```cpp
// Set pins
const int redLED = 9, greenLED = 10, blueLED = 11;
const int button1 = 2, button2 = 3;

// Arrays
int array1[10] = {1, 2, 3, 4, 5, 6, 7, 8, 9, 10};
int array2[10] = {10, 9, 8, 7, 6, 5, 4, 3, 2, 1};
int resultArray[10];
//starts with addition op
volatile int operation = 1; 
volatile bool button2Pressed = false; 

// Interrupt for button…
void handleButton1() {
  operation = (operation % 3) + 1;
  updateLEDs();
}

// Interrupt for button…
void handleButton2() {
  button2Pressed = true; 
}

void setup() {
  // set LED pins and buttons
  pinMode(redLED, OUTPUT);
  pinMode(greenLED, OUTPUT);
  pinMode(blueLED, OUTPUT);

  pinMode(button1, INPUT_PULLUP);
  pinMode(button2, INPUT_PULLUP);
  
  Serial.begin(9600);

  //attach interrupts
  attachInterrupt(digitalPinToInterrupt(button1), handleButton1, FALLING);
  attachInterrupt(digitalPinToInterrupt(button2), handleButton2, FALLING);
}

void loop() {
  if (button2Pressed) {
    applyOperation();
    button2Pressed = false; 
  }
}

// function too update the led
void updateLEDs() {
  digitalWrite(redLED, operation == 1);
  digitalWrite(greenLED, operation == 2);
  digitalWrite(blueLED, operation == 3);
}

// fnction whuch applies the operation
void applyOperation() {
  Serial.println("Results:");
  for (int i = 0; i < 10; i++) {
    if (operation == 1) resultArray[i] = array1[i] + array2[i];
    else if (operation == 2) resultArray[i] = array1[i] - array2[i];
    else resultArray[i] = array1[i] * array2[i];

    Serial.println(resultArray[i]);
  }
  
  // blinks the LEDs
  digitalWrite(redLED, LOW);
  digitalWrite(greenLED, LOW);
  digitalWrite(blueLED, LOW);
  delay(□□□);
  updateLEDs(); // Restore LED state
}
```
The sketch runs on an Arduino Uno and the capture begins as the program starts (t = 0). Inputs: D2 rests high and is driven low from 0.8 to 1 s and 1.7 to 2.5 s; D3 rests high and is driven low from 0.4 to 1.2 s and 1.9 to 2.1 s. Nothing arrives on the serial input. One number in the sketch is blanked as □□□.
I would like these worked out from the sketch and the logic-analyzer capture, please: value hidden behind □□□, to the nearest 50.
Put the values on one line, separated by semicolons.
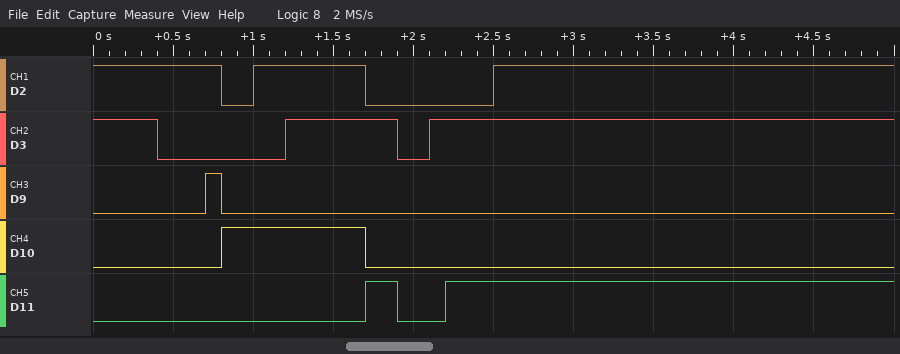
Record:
300
